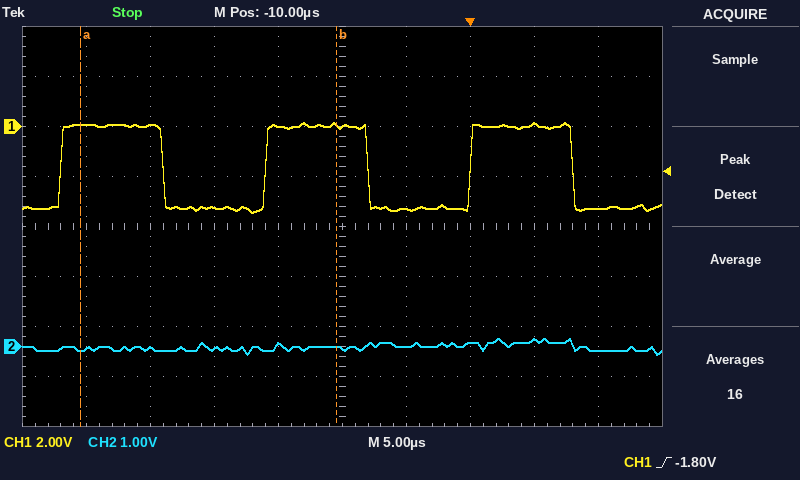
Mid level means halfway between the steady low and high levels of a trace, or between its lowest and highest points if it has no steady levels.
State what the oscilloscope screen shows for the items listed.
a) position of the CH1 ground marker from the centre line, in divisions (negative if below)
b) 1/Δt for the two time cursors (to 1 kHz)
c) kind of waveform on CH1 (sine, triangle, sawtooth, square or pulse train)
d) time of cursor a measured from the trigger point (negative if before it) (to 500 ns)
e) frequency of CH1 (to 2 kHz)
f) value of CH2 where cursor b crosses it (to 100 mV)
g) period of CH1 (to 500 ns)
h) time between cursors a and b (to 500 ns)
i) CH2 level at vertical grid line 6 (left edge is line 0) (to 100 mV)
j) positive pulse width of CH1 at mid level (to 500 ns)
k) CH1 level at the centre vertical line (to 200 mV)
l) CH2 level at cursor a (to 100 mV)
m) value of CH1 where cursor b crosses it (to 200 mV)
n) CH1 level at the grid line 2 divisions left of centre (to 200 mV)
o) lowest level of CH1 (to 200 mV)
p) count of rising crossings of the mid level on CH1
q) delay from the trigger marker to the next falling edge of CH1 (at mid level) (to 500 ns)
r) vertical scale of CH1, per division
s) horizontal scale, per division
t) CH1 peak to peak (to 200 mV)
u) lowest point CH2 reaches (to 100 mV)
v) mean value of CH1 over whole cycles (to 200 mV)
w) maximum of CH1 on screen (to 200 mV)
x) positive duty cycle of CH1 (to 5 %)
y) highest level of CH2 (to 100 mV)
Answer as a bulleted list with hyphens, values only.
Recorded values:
- +2.0 div
- 50 kHz
- square
- -30.5 µs
- 62 kHz
- 0.0 V
- 16.0 µs
- 20.0 µs
- 0.0 V
- 8.0 µs
- 0.0 V
- -100 mV
- 0.0 V
- -3.2 V
- -3.4 V
- 3
- 8.0 µs
- 2 V
- 5 µs
- 3.6 V
- -200 mV
- -1.6 V
- 200 mV
- 50 %
- 200 mV
